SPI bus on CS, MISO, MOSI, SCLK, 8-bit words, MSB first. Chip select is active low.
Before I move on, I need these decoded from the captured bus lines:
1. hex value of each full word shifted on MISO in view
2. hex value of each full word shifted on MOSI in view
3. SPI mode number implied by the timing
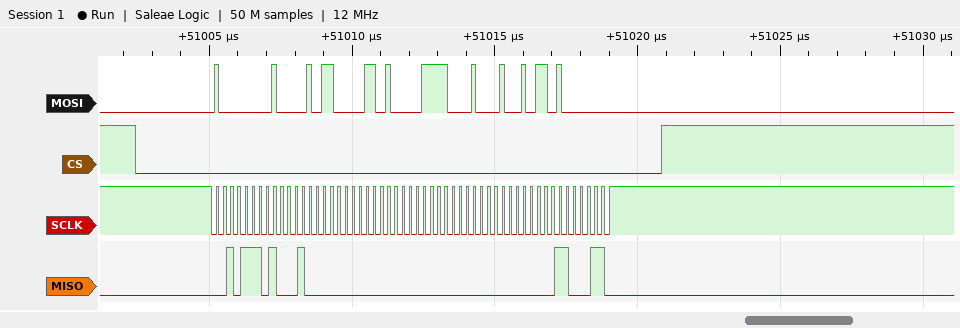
2E, 88, 00, 00, 00, 00, C6
80, 85, 86, 87, 88, 96, 80
3
